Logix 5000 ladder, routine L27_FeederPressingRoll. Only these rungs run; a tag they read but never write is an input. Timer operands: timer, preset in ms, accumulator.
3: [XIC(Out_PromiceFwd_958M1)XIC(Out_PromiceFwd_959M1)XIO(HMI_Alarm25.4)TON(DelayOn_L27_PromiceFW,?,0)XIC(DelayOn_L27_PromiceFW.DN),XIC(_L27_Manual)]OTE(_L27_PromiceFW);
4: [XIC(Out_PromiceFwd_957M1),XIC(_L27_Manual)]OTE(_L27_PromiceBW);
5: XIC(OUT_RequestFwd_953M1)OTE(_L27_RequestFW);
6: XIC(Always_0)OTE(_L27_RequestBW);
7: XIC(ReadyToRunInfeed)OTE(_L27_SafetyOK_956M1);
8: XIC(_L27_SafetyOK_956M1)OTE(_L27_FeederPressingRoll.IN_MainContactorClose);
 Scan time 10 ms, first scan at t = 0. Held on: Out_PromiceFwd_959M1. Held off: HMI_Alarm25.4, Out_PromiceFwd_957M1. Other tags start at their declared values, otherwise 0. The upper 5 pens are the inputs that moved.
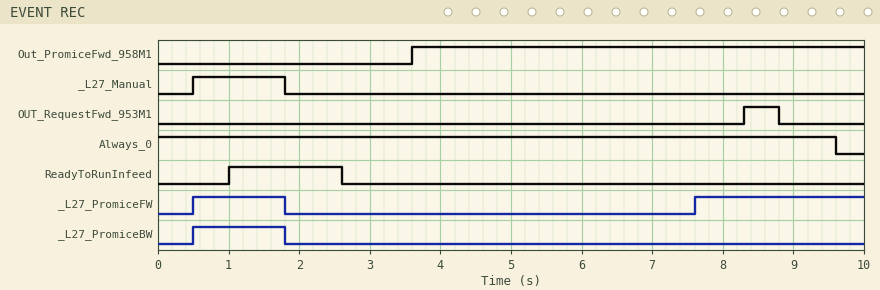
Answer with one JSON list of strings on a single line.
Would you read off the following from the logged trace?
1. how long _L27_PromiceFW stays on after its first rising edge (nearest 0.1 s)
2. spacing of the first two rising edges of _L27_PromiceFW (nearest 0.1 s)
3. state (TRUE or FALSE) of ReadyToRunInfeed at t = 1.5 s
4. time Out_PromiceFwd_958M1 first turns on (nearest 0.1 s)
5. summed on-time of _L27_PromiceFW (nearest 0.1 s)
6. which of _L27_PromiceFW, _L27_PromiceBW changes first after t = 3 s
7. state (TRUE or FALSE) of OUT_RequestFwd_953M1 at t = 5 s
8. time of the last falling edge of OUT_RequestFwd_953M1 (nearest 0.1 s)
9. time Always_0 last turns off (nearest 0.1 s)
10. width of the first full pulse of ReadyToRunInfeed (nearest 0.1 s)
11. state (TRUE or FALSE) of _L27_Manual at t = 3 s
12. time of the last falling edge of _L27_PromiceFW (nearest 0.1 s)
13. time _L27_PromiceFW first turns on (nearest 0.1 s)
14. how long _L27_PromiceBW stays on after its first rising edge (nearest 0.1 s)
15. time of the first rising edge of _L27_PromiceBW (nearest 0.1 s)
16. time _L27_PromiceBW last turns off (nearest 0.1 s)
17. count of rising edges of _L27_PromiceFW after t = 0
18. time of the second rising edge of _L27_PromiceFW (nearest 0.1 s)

["1.3 s", "7.1 s", "TRUE", "3.6 s", "3.7 s", "_L27_PromiceFW", "FALSE", "8.8 s", "9.6 s", "1.6 s", "FALSE", "1.8 s", "0.5 s", "1.3 s", "0.5 s", "1.8 s", "2", "7.6 s"]
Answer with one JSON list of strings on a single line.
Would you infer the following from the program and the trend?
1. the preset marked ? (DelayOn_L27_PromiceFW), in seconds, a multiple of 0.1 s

["4.0 s"]
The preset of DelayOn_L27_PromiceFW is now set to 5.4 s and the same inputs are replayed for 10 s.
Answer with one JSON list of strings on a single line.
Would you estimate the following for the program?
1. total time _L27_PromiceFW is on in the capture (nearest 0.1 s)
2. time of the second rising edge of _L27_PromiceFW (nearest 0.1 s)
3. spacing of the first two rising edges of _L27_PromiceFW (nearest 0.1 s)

["2.3 s", "9.0 s", "8.5 s"]
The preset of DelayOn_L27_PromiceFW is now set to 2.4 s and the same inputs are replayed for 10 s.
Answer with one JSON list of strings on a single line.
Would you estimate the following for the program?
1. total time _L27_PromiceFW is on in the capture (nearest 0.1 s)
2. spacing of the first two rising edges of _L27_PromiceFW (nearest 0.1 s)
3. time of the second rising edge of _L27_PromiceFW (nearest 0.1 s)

["5.3 s", "5.5 s", "6.0 s"]
